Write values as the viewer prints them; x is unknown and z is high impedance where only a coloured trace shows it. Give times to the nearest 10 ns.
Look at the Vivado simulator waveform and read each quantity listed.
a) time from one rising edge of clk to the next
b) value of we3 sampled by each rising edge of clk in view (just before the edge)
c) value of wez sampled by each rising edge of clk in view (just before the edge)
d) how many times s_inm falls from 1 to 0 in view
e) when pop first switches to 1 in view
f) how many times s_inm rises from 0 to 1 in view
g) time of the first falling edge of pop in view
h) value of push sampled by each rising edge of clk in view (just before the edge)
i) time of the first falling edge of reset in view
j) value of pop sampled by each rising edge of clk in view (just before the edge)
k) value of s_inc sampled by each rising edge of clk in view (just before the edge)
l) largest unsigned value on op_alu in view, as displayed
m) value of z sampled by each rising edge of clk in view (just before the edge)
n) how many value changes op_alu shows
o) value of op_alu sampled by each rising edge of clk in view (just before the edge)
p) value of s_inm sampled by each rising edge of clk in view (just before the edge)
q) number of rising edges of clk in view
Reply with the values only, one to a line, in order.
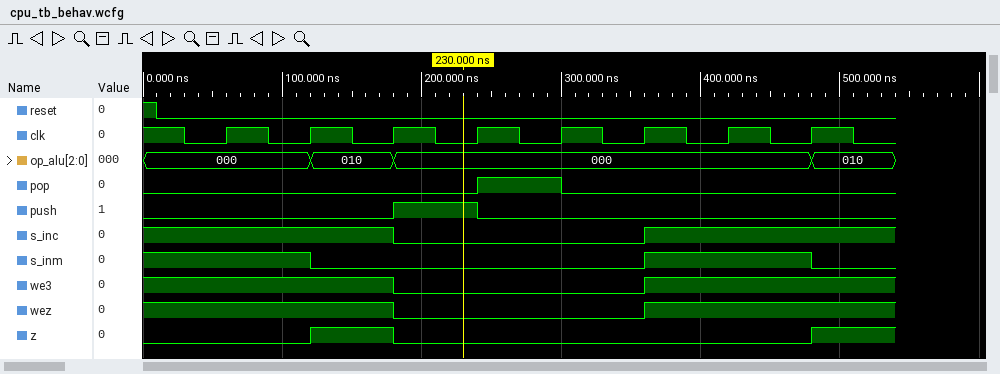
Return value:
60 ns
1 1 1 0 0 0 1 1
1 1 1 0 0 0 1 1
2
240 ns
1
300 ns
0 0 0 1 0 0 0 0
10 ns
0 0 0 0 1 0 0 0
1 1 1 0 0 0 1 1
010
0 0 1 0 0 0 0 0
3
000, 000, 010, 000, 000, 000, 000, 000
1 1 0 0 0 0 1 1
8
